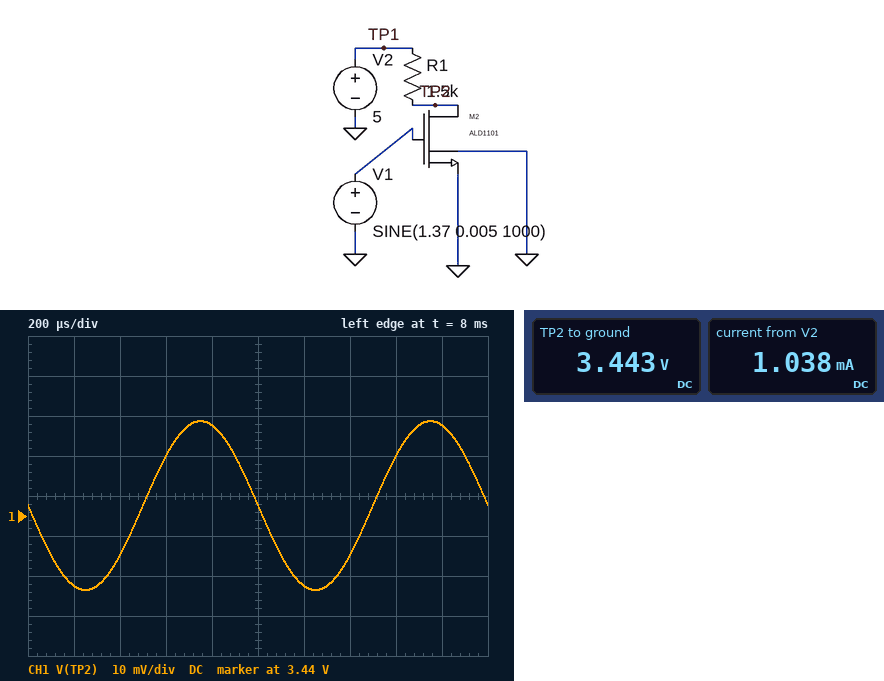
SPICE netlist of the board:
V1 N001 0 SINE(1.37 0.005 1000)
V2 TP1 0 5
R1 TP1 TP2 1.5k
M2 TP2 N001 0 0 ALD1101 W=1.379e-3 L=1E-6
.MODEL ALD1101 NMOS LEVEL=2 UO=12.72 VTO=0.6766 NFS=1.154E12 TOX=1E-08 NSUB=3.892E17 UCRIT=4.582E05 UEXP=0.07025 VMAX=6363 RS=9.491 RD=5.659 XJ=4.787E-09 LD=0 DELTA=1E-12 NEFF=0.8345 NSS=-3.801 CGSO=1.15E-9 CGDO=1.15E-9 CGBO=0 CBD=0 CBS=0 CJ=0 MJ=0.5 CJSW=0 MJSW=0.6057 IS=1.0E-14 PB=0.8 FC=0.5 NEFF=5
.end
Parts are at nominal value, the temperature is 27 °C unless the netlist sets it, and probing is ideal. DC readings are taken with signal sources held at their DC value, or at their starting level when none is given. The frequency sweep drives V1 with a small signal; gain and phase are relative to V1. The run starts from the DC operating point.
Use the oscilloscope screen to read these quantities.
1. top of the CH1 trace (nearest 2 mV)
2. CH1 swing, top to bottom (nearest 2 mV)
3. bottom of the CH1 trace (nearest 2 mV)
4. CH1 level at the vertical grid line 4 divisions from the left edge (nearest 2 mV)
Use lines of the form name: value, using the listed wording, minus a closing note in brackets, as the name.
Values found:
top of the CH1 trace: 3.464 V
CH1 swing, top to bottom: 42 mV
bottom of the CH1 trace: 3.422 V
CH1 level at the vertical grid line 4 divisions from the left edge: 3.462 V
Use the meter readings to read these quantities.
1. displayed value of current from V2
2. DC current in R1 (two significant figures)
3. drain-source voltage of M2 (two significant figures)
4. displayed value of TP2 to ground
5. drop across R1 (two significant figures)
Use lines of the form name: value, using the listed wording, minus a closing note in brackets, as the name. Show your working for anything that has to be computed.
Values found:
displayed value of current from V2: 1.038 mA
DC current in R1: (5 V - 3.443 V) / 1.5 kΩ = 1.0 mA
drain-source voltage of M2: 3.443 V = 3.4 V
displayed value of TP2 to ground: 3.443 V
drop across R1: 5 V - 3.443 V = 1.6 V
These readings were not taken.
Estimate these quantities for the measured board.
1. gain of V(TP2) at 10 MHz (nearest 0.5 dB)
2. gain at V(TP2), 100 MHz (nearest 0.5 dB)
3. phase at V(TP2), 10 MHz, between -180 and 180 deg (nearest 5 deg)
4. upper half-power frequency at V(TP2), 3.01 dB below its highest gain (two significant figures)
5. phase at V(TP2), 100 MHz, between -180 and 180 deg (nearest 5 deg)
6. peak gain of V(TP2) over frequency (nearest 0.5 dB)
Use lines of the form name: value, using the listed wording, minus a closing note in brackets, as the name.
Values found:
gain of V(TP2) at 10 MHz: 12.5 dB
gain at V(TP2), 100 MHz: 8.0 dB
phase at V(TP2), 10 MHz, between -180 and 180 deg: 170 deg
upper half-power frequency at V(TP2), 3.01 dB below its highest gain: 73 MHz
phase at V(TP2), 100 MHz, between -180 and 180 deg: 105 deg
peak gain of V(TP2) over frequency: 12.5 dB
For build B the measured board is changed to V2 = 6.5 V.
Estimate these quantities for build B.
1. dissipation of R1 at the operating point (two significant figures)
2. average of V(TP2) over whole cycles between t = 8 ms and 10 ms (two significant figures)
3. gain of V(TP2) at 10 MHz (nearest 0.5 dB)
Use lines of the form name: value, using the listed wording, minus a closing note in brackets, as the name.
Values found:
dissipation of R1 at the operating point: 1.7 mW
average of V(TP2) over whole cycles between t = 8 ms and 10 ms: 4.9 V
gain of V(TP2) at 10 MHz: 12.5 dB
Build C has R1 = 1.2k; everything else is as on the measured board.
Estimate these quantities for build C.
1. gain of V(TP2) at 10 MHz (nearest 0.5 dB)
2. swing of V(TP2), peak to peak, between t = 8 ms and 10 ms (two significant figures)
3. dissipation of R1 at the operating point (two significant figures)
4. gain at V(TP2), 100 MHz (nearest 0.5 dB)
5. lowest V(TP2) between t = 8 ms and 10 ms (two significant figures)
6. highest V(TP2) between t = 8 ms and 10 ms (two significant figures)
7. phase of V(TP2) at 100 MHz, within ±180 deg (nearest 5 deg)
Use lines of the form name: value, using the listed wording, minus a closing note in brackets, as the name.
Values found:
gain of V(TP2) at 10 MHz: 10.5 dB
swing of V(TP2), peak to peak, between t = 8 ms and 10 ms: 34 mV
dissipation of R1 at the operating point: 1.3 mW
gain at V(TP2), 100 MHz: 7.5 dB
lowest V(TP2) between t = 8 ms and 10 ms: 3.7 V
highest V(TP2) between t = 8 ms and 10 ms: 3.8 V
phase of V(TP2) at 100 MHz, within ±180 deg: 110 deg
